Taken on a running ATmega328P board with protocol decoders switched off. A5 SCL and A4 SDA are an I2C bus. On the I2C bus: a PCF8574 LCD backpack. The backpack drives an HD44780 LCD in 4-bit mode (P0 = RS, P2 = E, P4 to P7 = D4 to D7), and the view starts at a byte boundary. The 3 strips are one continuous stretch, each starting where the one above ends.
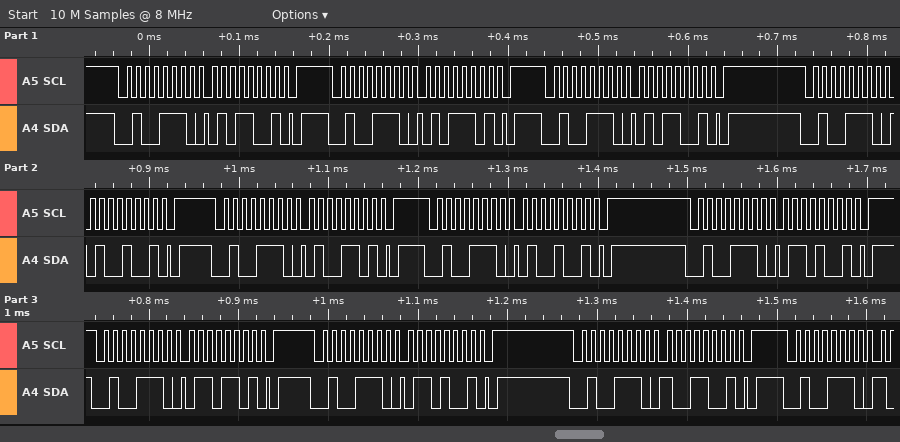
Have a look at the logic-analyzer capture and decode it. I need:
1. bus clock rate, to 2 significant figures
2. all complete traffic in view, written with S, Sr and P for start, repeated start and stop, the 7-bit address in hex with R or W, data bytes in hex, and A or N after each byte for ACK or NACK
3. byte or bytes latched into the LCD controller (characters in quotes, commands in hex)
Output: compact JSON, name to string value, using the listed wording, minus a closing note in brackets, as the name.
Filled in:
{"bus clock rate, to 2 significant figures": "100 kHz", "all complete traffic in view, written with S, Sr and P for start, repeated start and stop, the 7-bit address in hex with R or W, data bytes in hex, and A or N after each byte for ACK or NACK": "S 27W A 59 A P S 27W A 5D A P S 27W A 59 A P S 27W A 49 A P S 27W A 4D A P S 27W A 49 A P S 27W A 69 A P S 27W A 6D A P S 27W A 69 A P S 27W A 99 A P S 27W A", "byte or bytes latched into the LCD controller": "'T'"}
